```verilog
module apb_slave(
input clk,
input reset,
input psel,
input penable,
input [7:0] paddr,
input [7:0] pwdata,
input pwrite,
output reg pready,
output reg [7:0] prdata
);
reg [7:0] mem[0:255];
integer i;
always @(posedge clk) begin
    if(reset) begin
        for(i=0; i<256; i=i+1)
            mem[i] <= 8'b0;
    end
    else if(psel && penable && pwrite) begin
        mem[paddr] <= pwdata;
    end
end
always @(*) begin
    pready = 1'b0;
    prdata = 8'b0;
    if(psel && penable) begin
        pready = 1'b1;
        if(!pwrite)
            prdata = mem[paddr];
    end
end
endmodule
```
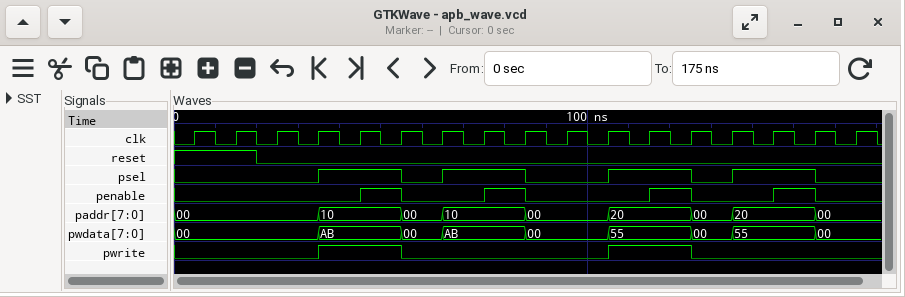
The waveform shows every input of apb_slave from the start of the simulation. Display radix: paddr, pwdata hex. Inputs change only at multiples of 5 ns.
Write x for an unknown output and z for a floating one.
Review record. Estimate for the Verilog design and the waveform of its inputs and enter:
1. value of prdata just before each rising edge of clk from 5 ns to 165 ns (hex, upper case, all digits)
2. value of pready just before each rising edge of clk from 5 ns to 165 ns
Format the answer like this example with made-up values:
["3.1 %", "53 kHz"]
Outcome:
["00, 00, 00, 00, 00, 00, 00, 00, AB, 00, 00, 00, 00, 00, 00, 55, 00", "0 0 0 0 0 1 0 0 1 0 0 0 1 0 0 1 0"]
